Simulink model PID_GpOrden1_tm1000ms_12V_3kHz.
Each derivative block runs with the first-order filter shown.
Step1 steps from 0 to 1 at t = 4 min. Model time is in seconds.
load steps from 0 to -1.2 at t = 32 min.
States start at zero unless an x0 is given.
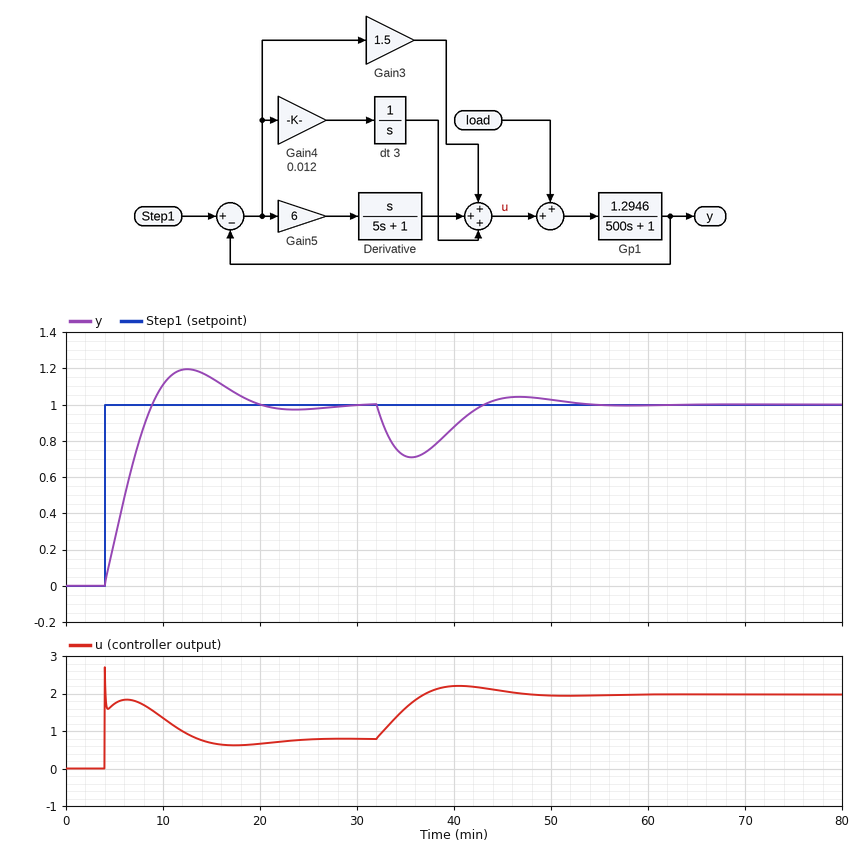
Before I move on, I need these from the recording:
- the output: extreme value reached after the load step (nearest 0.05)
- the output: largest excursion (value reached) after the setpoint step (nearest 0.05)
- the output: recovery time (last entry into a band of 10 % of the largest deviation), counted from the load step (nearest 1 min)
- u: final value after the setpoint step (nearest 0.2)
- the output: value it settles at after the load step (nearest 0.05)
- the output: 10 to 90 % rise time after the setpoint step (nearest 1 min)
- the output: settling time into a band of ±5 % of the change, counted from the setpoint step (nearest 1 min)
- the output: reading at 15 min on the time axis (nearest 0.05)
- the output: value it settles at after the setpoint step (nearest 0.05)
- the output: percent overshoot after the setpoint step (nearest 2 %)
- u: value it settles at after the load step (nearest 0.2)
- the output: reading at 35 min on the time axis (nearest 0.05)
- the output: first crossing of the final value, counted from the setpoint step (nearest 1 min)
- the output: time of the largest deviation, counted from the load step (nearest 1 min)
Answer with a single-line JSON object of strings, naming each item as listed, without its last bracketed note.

{"the output: extreme value reached after the load step": "0.70", "the output: largest excursion (value reached) after the setpoint step": "1.20", "the output: recovery time (last entry into a band of 10 % of the largest deviation), counted from the load step": "18 min", "u: final value after the setpoint step": "0.8", "the output: value it settles at after the load step": "1.00", "the output: 10 to 90 % rise time after the setpoint step": "4 min", "the output: settling time into a band of ±5 % of the change, counted from the setpoint step": "14 min", "the output: reading at 15 min on the time axis": "1.15", "the output: value it settles at after the setpoint step": "1.00", "the output: percent overshoot after the setpoint step": "20 %", "u: value it settles at after the load step": "2.0", "the output: reading at 35 min on the time axis": "0.70", "the output: first crossing of the final value, counted from the setpoint step": "5 min", "the output: time of the largest deviation, counted from the load step": "4 min"}
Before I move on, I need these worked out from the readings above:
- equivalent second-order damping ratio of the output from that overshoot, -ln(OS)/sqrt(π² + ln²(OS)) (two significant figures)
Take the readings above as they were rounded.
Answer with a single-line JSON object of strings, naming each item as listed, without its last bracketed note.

{"equivalent second-order damping ratio of the output from that overshoot, -ln(OS)/sqrt(π² + ln²(OS))": "0.46"}
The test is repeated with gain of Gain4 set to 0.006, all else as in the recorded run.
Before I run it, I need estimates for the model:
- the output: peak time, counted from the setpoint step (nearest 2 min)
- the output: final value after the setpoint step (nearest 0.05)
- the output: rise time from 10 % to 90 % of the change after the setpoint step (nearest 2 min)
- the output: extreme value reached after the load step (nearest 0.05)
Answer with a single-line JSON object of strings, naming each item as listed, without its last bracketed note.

{"the output: peak time, counted from the setpoint step": "12 min", "the output: final value after the setpoint step": "1.00", "the output: rise time from 10 % to 90 % of the change after the setpoint step": "6 min", "the output: extreme value reached after the load step": "0.65"}
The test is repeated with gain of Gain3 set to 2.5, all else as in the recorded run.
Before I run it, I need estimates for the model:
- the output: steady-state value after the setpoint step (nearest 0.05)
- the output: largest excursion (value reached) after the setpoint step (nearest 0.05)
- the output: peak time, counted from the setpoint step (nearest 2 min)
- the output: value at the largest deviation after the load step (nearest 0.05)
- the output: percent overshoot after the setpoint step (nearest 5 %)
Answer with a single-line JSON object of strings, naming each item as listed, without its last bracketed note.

{"the output: steady-state value after the setpoint step": "1.00", "the output: largest excursion (value reached) after the setpoint step": "1.10", "the output: peak time, counted from the setpoint step": "8 min", "the output: value at the largest deviation after the load step": "0.75", "the output: percent overshoot after the setpoint step": "10 %"}
